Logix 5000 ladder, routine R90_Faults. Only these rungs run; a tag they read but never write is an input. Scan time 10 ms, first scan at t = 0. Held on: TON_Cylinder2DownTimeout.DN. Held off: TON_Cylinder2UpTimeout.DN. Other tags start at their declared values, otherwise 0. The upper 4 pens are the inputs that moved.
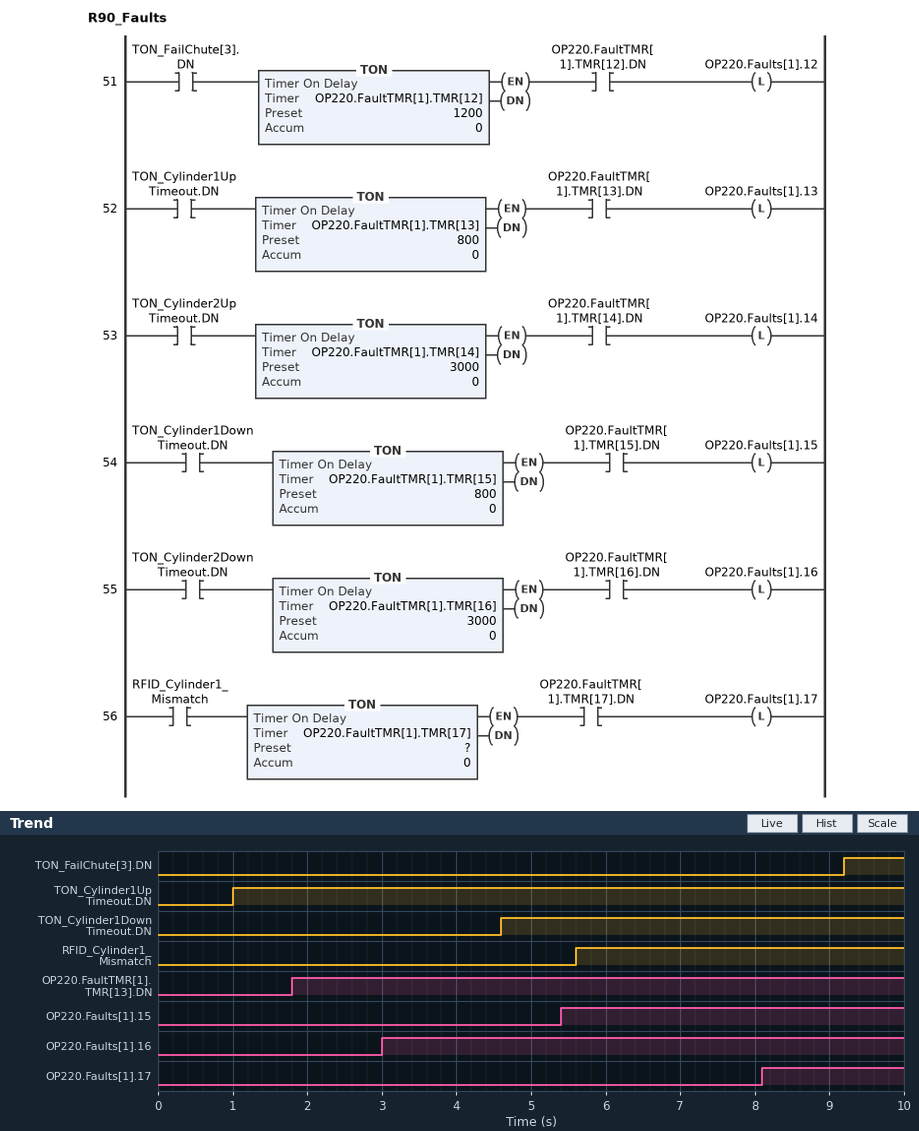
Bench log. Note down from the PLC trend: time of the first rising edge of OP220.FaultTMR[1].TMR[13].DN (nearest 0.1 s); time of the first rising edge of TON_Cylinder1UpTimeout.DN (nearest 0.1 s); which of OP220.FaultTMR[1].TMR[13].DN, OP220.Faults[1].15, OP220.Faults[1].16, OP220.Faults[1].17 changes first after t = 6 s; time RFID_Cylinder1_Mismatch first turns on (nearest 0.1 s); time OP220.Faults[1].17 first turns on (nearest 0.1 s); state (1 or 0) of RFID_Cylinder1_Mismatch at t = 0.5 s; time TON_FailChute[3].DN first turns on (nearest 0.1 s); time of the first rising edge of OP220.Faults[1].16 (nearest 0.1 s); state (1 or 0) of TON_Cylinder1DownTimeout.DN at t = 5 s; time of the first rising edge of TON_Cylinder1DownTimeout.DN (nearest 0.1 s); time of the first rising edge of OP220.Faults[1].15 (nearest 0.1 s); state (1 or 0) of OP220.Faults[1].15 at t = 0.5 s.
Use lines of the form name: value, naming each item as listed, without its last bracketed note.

time of the first rising edge of OP220.FaultTMR[1].TMR[13].DN: 1.8 s
time of the first rising edge of TON_Cylinder1UpTimeout.DN: 1.0 s
which of OP220.FaultTMR[1].TMR[13].DN, OP220.Faults[1].15, OP220.Faults[1].16, OP220.Faults[1].17 changes first after t = 6 s: OP220.Faults[1].17
time RFID_Cylinder1_Mismatch first turns on: 5.6 s
time OP220.Faults[1].17 first turns on: 8.1 s
state (1 or 0) of RFID_Cylinder1_Mismatch at t = 0.5 s: 0
time TON_FailChute[3].DN first turns on: 9.2 s
time of the first rising edge of OP220.Faults[1].16: 3.0 s
state (1 or 0) of TON_Cylinder1DownTimeout.DN at t = 5 s: 1
time of the first rising edge of TON_Cylinder1DownTimeout.DN: 4.6 s
time of the first rising edge of OP220.Faults[1].15: 5.4 s
state (1 or 0) of OP220.Faults[1].15 at t = 0.5 s: 0
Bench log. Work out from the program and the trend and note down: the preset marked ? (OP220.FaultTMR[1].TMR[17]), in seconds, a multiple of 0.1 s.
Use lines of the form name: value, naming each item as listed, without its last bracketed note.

the preset marked ? (OP220.FaultTMR[1].TMR[17]), in seconds, a multiple of 0.1 s: 2.5 s
